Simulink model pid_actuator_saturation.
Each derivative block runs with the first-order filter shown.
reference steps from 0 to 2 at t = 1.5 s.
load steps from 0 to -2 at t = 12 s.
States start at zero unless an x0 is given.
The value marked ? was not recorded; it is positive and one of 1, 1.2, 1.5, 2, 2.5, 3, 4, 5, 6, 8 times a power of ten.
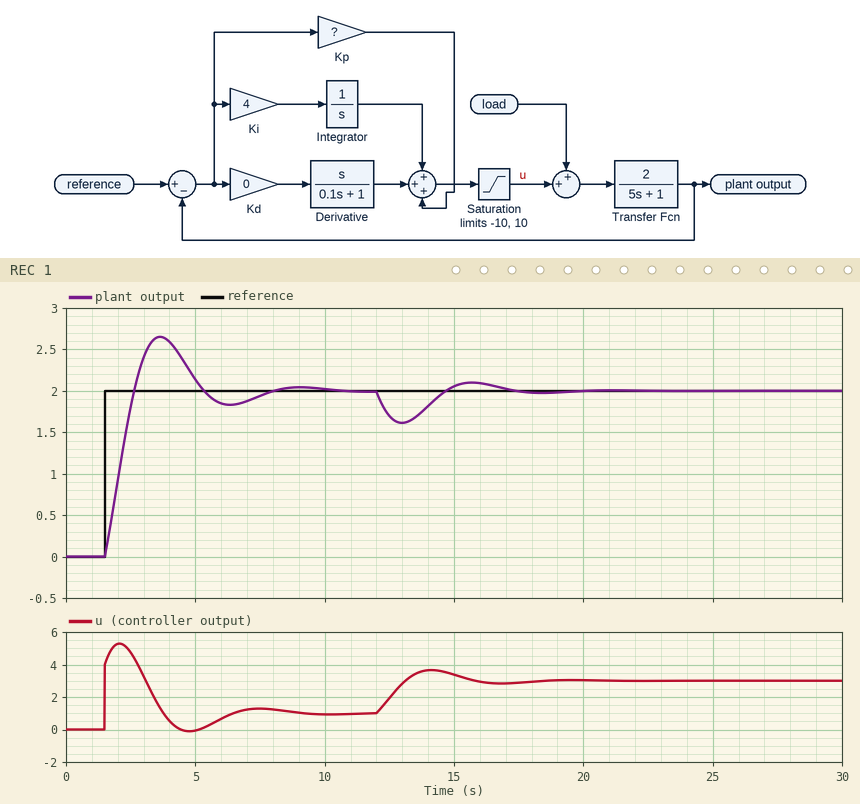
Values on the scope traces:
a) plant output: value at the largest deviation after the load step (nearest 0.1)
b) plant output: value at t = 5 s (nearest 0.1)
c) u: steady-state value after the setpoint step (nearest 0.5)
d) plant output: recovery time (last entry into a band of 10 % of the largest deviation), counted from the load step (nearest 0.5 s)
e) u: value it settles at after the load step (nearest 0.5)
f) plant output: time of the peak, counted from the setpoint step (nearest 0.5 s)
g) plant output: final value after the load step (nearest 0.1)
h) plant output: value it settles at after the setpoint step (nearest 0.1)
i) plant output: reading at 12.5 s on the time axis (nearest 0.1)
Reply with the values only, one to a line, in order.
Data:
1.6
2.1
1.0
5.0 s
3.0
2.0 s
2.0
2.0
1.7
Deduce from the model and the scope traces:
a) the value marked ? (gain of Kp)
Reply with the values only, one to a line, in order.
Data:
2
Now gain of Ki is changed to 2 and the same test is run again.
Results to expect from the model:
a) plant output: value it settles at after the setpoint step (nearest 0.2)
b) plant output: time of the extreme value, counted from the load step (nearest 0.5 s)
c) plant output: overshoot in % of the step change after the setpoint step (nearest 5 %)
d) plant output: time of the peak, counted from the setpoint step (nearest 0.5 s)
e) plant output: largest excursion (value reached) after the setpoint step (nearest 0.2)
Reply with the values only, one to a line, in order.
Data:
2.0
1.5 s
20 %
3.0 s
2.4
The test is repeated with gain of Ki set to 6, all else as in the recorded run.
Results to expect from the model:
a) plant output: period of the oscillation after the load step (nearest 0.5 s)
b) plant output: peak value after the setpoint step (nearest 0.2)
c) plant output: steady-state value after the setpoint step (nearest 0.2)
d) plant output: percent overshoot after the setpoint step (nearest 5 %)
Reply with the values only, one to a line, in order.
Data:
4.5 s
2.8
2.0
40 %
